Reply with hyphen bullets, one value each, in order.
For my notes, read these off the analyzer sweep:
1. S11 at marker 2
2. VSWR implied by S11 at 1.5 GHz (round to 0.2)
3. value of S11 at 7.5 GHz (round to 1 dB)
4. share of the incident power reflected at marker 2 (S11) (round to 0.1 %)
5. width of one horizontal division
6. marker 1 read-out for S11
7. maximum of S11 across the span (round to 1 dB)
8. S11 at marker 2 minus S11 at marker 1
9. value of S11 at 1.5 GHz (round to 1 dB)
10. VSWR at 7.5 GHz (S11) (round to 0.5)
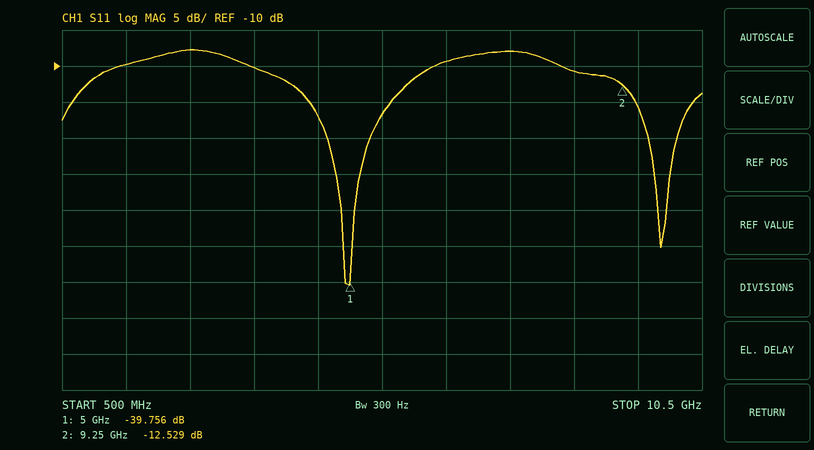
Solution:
- -12.529 dB
- 2.0
- -8 dB
- 5.6 %
- 1 GHz
- -39.756 dB
- -8 dB
- 27.227 dB
- -10 dB
- 2.5
